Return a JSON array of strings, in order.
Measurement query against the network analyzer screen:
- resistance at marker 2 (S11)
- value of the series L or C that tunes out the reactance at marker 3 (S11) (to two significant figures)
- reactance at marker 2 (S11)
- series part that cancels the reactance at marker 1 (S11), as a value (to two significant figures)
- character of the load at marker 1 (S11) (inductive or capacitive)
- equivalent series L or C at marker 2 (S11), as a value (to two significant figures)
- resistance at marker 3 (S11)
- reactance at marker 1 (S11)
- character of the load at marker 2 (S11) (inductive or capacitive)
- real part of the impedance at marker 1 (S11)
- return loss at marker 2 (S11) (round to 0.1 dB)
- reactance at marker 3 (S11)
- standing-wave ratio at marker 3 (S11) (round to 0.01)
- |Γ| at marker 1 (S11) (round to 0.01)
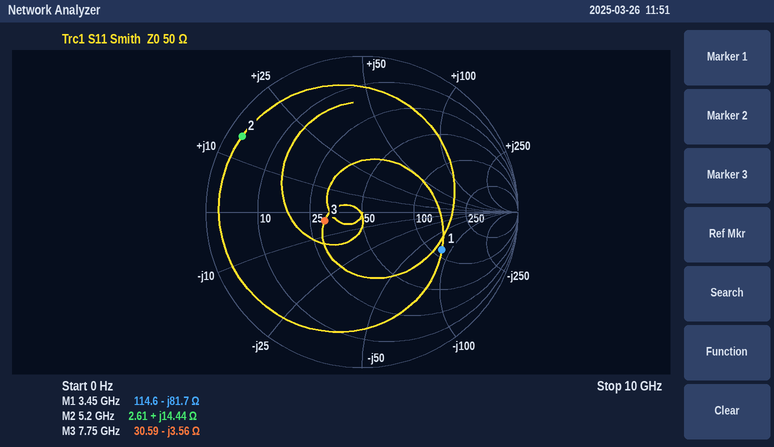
["2.61 Ω", "73 pH", "+14.44 Ω", "3.8 nH", "capacitive", "440 pH", "30.59 Ω", "-81.7 Ω", "inductive", "114.6 Ω", "0.8 dB", "-3.56 Ω", "1.65", "0.57"]
